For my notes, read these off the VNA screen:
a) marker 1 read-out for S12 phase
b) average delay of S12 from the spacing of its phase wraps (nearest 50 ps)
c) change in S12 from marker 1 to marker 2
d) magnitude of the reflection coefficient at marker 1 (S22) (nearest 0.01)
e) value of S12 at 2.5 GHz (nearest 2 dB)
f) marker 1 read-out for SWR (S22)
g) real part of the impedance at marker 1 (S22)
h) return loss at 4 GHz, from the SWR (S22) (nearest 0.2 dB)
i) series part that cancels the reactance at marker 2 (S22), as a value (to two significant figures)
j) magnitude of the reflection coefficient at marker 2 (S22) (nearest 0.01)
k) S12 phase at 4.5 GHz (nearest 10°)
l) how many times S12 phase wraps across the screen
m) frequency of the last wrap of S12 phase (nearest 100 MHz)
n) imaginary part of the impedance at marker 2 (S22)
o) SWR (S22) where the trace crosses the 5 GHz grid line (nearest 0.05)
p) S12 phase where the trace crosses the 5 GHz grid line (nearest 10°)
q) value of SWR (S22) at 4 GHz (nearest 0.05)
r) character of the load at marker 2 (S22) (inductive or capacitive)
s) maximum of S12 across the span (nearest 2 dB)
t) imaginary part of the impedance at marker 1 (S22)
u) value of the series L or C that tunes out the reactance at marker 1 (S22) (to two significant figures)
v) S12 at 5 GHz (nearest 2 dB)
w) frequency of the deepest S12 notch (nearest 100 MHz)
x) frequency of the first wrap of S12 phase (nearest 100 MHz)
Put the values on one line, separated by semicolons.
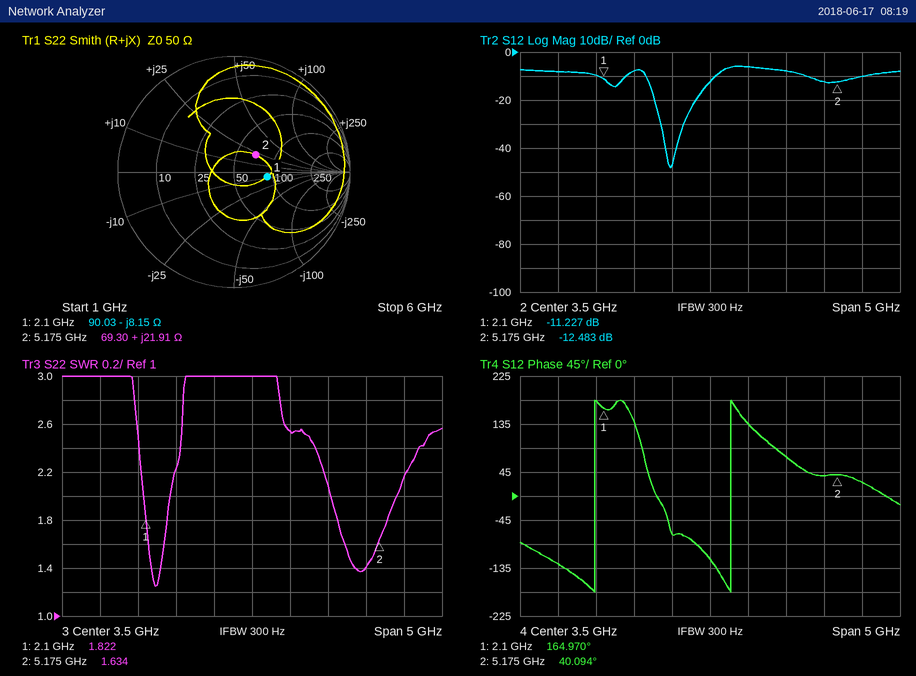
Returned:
164.970°; 550 ps; -1.256 dB; 0.29; -8 dB; 1.822; 90.03 Ω; 7.2 dB; 1.4 pF; 0.24; 70°; 2; 3.8 GHz; +21.91 Ω; 1.40; 40°; 2.55; inductive; -6 dB; -8.15 Ω; 620 pH; -12 dB; 3.0 GHz; 2.0 GHz
